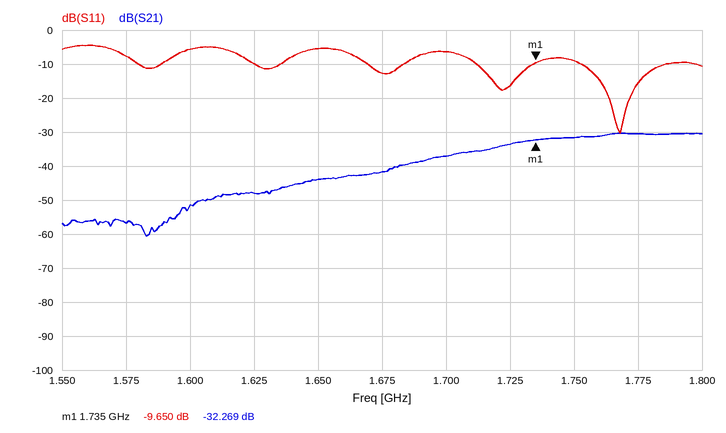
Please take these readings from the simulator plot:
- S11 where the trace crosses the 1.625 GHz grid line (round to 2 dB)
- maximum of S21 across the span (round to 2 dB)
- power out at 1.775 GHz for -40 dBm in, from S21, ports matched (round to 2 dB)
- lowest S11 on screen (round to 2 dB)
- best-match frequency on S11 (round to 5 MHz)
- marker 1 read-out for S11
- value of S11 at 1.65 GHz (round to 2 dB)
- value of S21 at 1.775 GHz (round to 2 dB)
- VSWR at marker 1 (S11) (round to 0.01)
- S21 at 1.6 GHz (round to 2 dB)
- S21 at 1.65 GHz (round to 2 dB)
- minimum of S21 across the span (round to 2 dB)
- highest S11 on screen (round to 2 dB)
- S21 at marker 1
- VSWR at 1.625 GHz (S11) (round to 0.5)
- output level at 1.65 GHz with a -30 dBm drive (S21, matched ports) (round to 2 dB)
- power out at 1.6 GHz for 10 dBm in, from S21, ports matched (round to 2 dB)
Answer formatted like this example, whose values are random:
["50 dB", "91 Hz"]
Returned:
["-10 dB", "-30 dB", "-70 dBm", "-30 dB", "1.770 GHz", "-9.650 dB", "-6 dB", "-30 dB", "1.98", "-52 dB", "-44 dB", "-60 dB", "-4 dB", "-32.269 dB", "2.0", "-74 dBm", "-42 dBm"]
